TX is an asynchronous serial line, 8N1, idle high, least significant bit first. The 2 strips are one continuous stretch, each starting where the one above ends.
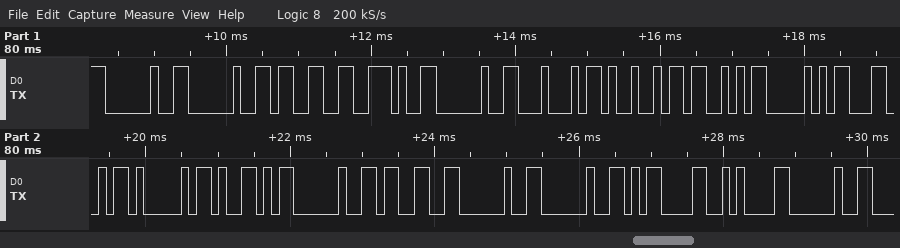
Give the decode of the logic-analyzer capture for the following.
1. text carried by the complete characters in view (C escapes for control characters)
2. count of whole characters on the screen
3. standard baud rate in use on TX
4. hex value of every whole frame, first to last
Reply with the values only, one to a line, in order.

"  3. DISPLAY 3  \r\n "
19
9600 baud
20 20 33 2E 20 44 49 53 50 4C 41 59 20 33 20 20 0D 0A 20
